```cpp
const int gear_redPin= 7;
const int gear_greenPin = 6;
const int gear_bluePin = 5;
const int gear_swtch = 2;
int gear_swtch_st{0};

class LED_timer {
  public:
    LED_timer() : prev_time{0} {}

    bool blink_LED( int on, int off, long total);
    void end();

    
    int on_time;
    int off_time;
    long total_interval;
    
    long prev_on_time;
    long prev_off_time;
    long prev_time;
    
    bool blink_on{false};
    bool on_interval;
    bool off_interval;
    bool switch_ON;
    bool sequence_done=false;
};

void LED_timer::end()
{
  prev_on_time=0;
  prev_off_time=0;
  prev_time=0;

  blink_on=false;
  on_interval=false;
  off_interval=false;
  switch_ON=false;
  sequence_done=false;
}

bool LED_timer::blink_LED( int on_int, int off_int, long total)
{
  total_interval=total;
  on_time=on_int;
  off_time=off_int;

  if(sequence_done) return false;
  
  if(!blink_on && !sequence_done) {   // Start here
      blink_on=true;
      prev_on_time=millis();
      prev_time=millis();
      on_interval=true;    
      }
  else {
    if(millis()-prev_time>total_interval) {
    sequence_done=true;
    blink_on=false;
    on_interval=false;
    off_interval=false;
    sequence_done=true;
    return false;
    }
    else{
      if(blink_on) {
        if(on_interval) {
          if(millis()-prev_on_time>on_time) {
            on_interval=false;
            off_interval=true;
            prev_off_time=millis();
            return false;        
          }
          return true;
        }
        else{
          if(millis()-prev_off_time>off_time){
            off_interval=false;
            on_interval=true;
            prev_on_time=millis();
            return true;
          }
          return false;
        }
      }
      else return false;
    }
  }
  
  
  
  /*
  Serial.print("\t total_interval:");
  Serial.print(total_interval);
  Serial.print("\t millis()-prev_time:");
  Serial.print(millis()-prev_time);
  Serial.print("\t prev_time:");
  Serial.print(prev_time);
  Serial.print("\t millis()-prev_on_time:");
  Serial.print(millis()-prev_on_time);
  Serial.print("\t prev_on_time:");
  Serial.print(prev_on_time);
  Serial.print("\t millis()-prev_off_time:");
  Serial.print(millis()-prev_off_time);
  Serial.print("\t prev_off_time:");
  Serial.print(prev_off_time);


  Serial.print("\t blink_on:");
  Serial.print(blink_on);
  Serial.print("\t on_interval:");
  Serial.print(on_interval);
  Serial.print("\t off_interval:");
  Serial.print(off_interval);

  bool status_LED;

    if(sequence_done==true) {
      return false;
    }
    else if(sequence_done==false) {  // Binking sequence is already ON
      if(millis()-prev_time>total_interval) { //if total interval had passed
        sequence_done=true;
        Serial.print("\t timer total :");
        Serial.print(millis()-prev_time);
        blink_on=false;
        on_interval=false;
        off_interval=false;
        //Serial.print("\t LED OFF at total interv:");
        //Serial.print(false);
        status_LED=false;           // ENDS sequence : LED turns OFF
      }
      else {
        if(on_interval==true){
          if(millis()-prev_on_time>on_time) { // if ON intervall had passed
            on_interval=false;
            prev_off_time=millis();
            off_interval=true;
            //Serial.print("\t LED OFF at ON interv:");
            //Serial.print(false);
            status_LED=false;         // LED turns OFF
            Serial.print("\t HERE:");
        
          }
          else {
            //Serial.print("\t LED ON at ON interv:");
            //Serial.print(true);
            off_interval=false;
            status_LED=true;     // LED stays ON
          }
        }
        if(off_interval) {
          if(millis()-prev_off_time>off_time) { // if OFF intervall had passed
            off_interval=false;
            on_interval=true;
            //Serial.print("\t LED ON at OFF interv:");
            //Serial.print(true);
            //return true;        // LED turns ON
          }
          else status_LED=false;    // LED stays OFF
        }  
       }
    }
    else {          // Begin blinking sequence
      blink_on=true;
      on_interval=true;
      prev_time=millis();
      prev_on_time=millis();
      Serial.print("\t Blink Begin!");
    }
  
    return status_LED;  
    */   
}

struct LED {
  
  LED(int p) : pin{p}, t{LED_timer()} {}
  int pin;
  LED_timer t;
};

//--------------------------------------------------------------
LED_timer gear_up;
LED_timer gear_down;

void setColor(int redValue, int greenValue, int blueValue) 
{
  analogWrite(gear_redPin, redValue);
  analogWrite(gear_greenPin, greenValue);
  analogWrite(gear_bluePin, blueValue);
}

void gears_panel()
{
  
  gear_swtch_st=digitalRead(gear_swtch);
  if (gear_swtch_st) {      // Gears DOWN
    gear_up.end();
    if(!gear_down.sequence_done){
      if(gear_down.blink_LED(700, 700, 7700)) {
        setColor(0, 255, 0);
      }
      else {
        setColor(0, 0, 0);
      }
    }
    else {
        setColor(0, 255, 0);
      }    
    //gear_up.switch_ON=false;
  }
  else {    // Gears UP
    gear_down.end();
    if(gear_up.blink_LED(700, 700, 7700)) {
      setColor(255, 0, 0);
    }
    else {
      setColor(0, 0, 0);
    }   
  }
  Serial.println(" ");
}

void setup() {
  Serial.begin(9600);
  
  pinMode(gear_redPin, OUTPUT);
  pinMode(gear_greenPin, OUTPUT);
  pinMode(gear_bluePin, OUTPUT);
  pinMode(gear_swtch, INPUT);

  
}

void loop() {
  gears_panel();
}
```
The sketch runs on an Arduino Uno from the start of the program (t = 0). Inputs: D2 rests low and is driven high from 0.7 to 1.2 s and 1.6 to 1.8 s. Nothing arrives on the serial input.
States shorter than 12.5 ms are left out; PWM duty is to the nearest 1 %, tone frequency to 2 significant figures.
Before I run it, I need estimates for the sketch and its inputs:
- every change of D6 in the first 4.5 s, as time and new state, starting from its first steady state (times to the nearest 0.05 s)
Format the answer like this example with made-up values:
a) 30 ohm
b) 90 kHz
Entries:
a) 0 s low; 0.7 s high; 1.2 s low; 1.6 s high; 1.8 s low
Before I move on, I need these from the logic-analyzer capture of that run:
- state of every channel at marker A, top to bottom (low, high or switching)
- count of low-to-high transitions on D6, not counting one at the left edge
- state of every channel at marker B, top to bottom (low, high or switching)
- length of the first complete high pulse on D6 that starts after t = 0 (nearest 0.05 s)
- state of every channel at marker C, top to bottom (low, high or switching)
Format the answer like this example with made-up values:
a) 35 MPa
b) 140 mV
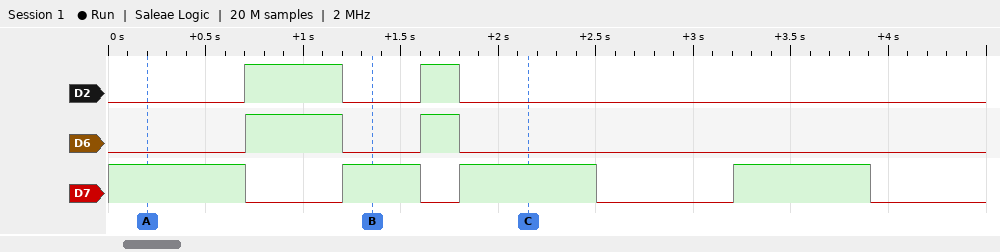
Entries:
a) D2 low, D6 low, D7 high
b) 2
c) D2 low, D6 low, D7 high
d) 0.50 s
e) D2 low, D6 low, D7 high
